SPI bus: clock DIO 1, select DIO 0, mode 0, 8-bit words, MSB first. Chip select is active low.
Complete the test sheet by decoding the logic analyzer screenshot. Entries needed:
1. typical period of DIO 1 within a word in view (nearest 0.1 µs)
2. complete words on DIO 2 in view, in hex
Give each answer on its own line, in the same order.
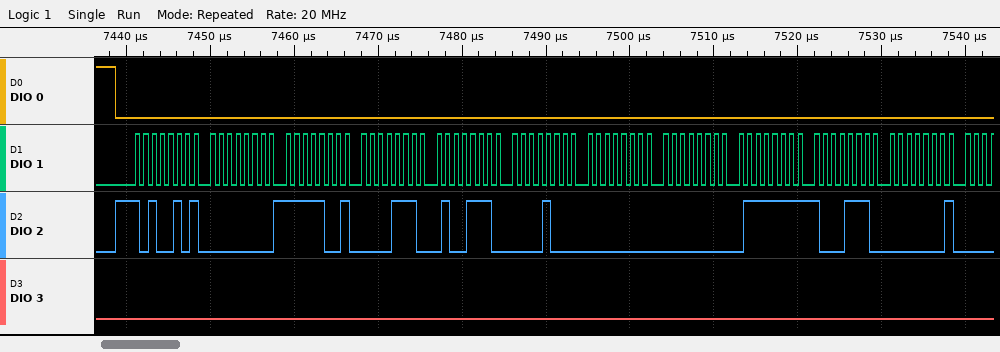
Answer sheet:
1 µs
A5, 00, F9, 0E, 4E, 08, 00, 00, 7F, 8E, 01
